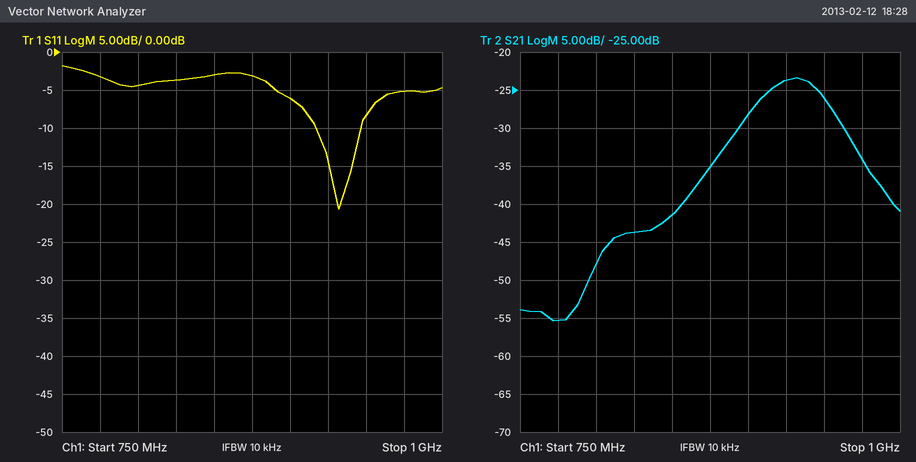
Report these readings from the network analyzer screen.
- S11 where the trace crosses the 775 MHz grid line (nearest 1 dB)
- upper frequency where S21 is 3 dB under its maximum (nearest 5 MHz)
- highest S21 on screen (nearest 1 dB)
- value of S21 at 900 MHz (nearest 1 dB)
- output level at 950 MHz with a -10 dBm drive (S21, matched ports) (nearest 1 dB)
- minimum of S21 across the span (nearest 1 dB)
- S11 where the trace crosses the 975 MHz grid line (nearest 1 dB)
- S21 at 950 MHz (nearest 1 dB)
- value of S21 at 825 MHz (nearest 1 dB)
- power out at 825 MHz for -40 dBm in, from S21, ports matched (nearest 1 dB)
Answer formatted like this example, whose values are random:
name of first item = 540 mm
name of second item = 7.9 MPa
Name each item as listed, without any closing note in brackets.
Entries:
S11 where the trace crosses the 775 MHz grid line = -3 dB
upper frequency where S21 is 3 dB under its maximum = 950 MHz
highest S21 on screen = -23 dB
value of S21 at 900 MHz = -28 dB
output level at 950 MHz with a -10 dBm drive (S21, matched ports) = -36 dBm
minimum of S21 across the span = -55 dB
S11 where the trace crosses the 975 MHz grid line = -5 dB
S21 at 950 MHz = -26 dB
value of S21 at 825 MHz = -44 dB
power out at 825 MHz for -40 dBm in, from S21, ports matched = -84 dBm
